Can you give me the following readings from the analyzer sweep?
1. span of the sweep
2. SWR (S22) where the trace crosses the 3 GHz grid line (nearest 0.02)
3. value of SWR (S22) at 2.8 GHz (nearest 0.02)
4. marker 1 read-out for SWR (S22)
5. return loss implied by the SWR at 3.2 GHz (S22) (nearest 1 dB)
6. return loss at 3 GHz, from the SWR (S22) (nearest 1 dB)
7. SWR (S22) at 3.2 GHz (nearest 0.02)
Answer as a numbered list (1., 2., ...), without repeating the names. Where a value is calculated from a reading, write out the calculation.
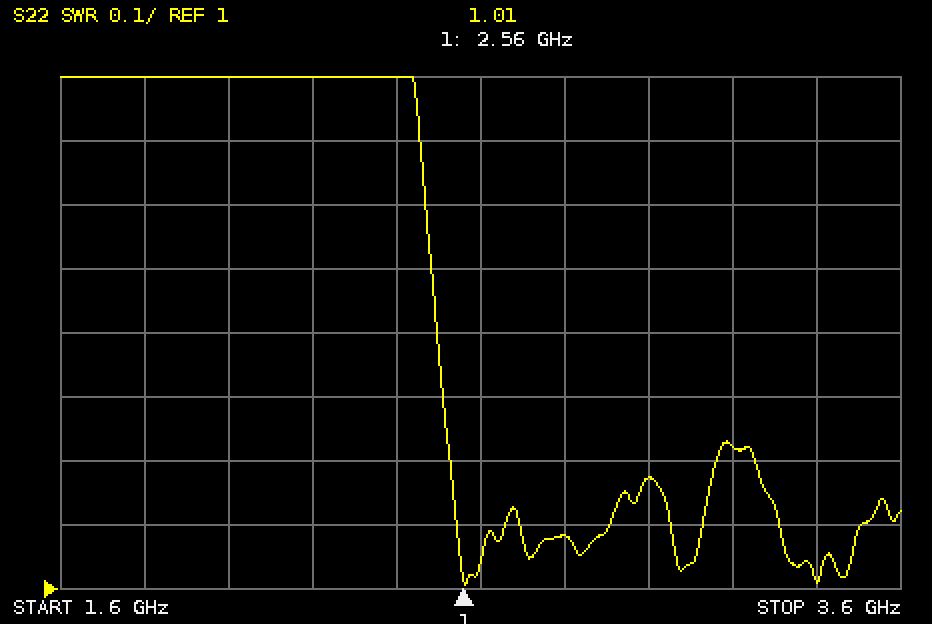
1. 2 GHz
2. 1.18
3. 1.08
4. 1.01
5. −20 log10((1.22 − 1)/(1.22 + 1)) ≈ 20 dB
6. −20 log10((1.18 − 1)/(1.18 + 1)) ≈ 22 dB
7. 1.22
